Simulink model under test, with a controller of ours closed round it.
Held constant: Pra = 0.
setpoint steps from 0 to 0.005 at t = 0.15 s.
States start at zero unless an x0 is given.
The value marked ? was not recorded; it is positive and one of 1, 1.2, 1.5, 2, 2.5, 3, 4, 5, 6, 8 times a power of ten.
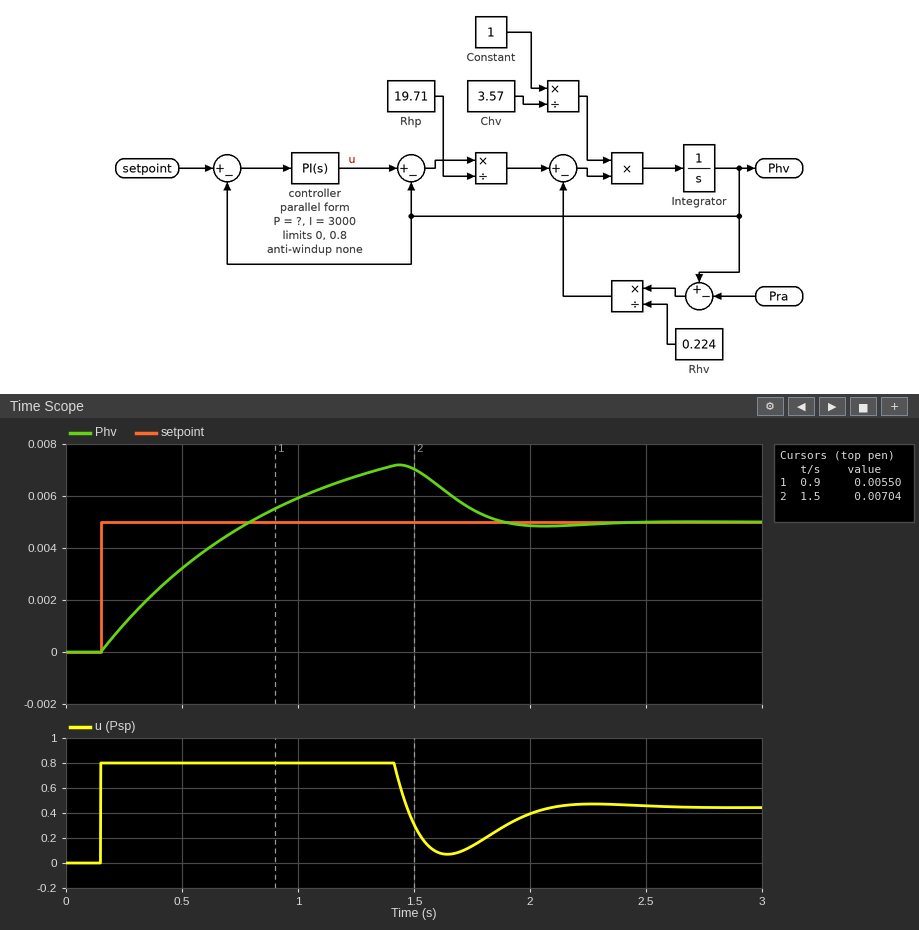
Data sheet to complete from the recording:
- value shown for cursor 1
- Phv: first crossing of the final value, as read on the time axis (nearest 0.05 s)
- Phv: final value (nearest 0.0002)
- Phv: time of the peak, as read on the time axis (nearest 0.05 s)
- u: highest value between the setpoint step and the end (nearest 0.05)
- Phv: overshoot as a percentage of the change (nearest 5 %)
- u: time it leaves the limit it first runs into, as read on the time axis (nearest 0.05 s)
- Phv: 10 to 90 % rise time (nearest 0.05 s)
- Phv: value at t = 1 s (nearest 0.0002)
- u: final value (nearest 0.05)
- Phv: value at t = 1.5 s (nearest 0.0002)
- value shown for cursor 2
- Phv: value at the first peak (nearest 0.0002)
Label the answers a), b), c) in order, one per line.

a) 0.00550
b) 0.80 s
c) 0.0050
d) 1.45 s
e) 0.80
f) 45 %
g) 1.40 s
h) 0.50 s
i) 0.0060
j) 0.45
k) 0.0070
l) 0.00704
m) 0.0072
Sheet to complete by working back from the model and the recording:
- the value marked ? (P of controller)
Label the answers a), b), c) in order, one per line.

a) 500
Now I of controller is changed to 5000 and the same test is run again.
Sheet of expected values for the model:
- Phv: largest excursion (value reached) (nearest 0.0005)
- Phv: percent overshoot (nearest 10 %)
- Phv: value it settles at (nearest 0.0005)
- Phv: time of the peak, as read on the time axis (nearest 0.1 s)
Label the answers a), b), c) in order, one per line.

a) 0.0075
b) 50 %
c) 0.0050
d) 1.5 s
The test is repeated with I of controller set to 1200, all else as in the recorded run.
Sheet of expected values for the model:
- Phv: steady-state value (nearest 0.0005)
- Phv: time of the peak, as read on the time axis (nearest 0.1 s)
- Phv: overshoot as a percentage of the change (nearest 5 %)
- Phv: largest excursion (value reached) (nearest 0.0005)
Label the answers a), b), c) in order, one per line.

a) 0.0050
b) 1.2 s
c) 30 %
d) 0.0065
